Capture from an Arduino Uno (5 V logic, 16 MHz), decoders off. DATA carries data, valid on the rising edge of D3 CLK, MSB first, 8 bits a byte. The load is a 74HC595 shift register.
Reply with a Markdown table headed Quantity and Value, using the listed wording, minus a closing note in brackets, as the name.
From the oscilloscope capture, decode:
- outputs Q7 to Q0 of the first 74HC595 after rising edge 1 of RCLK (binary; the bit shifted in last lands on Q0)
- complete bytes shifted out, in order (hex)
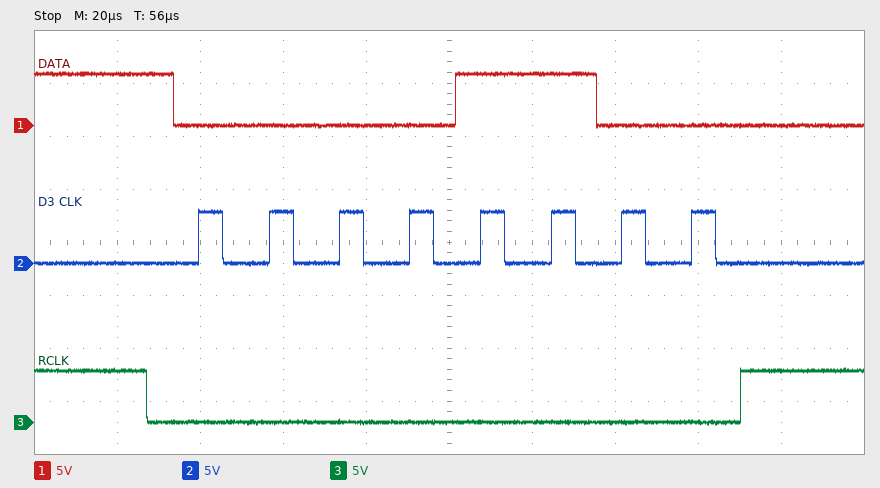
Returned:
| Quantity | Value |
|---|---|
| outputs Q7 to Q0 of the first 74HC595 after rising edge 1 of RCLK | 00001100 |
| complete bytes shifted out, in order | 0C |
